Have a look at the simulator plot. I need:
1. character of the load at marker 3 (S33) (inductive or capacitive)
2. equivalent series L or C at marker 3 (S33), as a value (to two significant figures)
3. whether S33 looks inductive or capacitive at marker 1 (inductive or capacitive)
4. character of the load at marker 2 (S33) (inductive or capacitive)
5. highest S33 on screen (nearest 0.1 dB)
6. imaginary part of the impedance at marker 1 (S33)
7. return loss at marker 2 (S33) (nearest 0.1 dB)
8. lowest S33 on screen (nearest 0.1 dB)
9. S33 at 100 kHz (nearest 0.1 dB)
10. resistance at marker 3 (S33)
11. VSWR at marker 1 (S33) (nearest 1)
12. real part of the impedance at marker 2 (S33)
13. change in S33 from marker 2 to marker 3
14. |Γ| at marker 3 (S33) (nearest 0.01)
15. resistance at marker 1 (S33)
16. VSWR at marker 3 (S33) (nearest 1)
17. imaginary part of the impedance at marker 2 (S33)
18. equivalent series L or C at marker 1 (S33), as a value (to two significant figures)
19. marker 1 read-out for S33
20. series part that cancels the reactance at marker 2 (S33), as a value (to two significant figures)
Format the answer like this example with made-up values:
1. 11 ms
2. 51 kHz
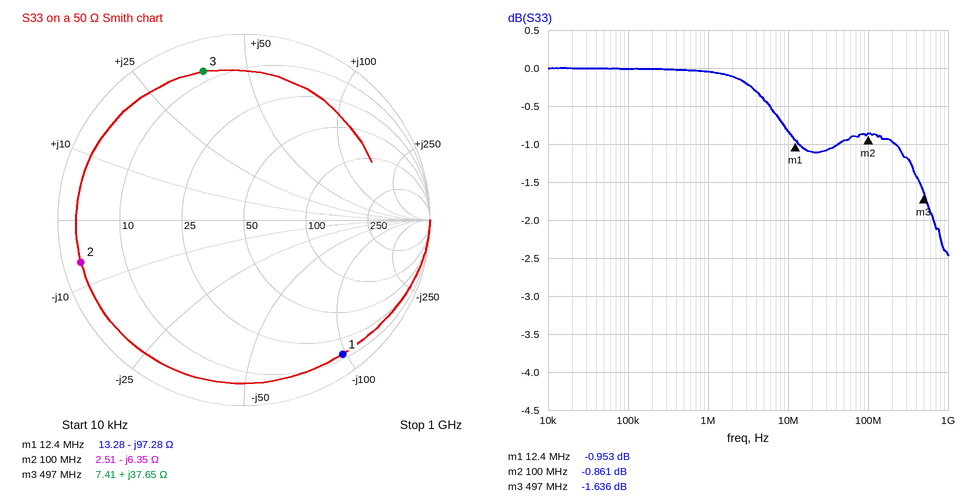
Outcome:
1. inductive
2. 12 nH
3. capacitive
4. capacitive
5. 0.0 dB
6. -97.28 Ω
7. 0.9 dB
8. -2.5 dB
9. 0.0 dB
10. 7.41 Ω
11. 18
12. 2.51 Ω
13. -0.775 dB
14. 0.83
15. 13.28 Ω
16. 11
17. -6.35 Ω
18. 130 pF
19. -0.953 dB
20. 10 nH
